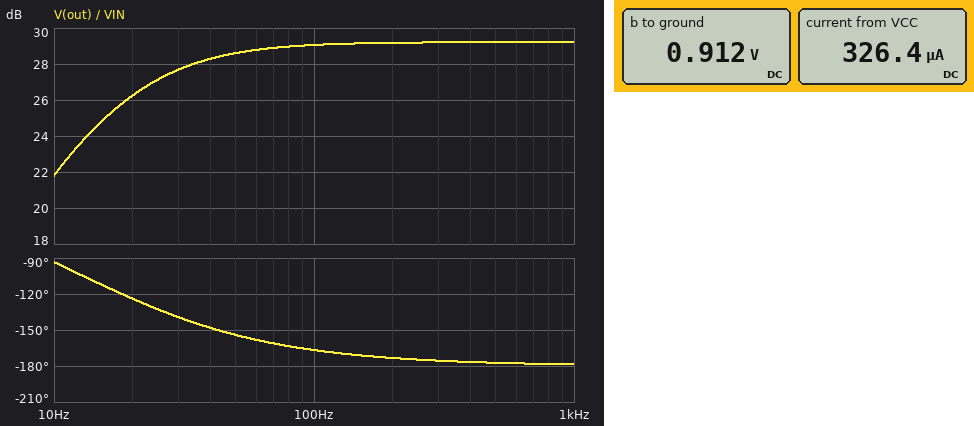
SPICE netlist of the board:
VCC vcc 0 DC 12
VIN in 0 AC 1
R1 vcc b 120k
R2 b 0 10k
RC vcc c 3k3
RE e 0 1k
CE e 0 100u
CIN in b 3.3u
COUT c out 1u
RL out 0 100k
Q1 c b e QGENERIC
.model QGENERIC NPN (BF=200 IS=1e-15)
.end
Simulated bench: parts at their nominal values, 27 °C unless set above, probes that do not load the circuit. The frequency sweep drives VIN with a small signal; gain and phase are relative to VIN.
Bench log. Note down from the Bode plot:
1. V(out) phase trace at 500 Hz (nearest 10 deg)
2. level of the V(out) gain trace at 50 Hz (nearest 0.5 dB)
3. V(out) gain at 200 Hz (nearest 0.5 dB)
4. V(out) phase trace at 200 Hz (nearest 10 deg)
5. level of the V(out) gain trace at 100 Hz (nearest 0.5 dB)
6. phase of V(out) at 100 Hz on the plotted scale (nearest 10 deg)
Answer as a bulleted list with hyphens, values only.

- -180 deg
- 28.5 dB
- 29.0 dB
- -170 deg
- 29.0 dB
- -170 deg
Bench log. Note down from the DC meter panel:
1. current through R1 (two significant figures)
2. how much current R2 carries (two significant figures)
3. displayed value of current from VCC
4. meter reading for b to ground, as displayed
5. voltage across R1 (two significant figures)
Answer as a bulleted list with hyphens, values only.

- 92 µA
- 91 µA
- 326.4 µA
- 0.912 V
- 11 V
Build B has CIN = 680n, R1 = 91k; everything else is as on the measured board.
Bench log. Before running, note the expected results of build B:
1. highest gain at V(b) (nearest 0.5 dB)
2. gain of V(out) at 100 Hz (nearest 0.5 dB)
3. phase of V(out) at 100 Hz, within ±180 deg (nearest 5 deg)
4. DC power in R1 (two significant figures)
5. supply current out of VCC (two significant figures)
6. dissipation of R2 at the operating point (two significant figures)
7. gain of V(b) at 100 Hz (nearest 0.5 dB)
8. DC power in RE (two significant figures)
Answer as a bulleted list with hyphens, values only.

- 0 dB
- 33.5 dB
- -140 deg
- 1.3 mW
- 590 µA
- 140 µW
- -1.0 dB
- 220 µW
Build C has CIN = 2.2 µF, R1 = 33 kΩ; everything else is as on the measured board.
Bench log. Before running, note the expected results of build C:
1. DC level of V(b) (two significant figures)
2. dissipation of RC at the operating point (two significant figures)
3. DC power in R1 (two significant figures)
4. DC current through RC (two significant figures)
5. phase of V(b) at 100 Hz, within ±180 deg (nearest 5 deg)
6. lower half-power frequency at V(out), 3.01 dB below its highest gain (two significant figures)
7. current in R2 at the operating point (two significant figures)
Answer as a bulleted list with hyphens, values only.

- 2.7 V
- 13 mW
- 2.6 mW
- 2.0 mA
- 10 deg
- 150 Hz
- 270 µA
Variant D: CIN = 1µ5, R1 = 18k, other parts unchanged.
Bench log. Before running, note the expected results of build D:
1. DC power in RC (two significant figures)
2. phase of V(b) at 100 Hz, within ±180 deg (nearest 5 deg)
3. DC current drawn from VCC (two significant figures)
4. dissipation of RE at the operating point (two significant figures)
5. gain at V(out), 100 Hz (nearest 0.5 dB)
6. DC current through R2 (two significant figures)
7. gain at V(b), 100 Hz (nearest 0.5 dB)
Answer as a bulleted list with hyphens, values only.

- 25 mW
- 45 deg
- 3.2 mA
- 8.1 mW
- -12.5 dB
- 360 µA
- -32.5 dB
